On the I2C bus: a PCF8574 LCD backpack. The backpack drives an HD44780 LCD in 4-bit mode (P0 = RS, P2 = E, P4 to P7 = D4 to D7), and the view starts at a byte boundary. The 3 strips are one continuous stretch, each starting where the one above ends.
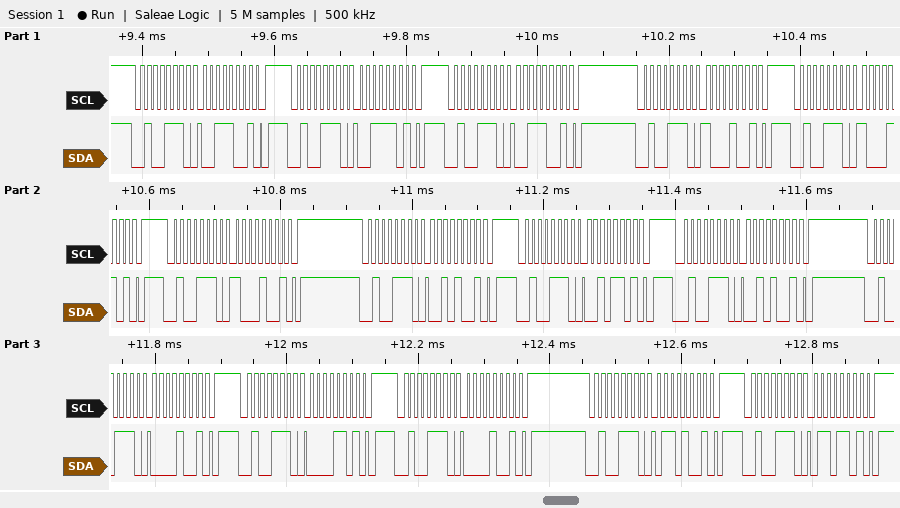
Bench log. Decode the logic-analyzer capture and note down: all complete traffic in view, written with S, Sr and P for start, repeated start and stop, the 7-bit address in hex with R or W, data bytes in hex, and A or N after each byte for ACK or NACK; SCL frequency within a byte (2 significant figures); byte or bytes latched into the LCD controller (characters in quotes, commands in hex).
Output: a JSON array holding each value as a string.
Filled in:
["S 27W A 39 A P S 27W A 3D A P S 27W A 39 A P S 27W A 89 A P S 27W A 8D A P S 27W A 89 A P S 27W A 29 A P S 27W A 2D A P S 27W A 29 A P S 27W A 09 A P S 27W A 0D A P S 27W A 09 A P S 27W A 69 A P S 27W A 6D A P", "100 kHz", "'8' ' '"]
